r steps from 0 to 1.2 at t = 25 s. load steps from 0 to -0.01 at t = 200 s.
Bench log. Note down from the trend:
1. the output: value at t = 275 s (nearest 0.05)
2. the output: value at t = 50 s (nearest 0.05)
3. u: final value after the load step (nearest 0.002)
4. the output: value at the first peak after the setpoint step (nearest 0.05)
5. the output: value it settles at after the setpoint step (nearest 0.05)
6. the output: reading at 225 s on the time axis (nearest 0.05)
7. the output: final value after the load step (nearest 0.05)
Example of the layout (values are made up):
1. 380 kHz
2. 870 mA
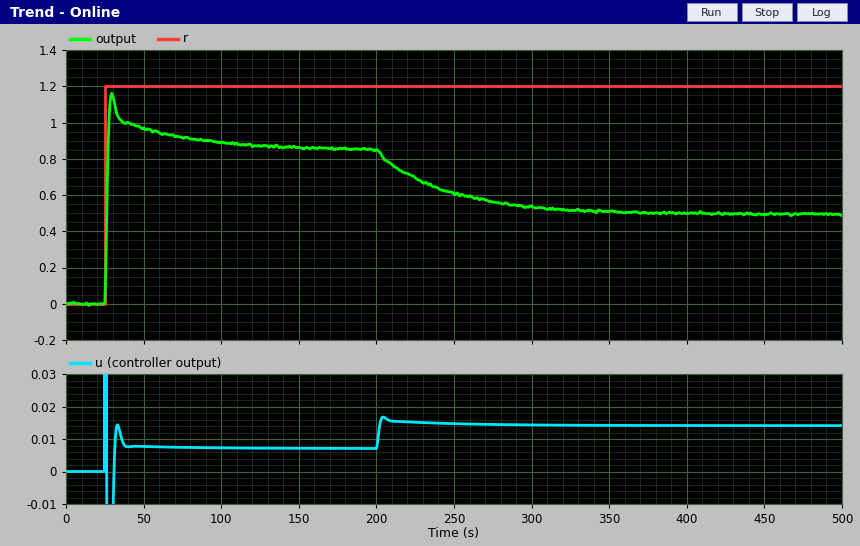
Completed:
1. 0.55
2. 0.95
3. 0.014
4. 1.15
5. 0.85
6. 0.70
7. 0.50
